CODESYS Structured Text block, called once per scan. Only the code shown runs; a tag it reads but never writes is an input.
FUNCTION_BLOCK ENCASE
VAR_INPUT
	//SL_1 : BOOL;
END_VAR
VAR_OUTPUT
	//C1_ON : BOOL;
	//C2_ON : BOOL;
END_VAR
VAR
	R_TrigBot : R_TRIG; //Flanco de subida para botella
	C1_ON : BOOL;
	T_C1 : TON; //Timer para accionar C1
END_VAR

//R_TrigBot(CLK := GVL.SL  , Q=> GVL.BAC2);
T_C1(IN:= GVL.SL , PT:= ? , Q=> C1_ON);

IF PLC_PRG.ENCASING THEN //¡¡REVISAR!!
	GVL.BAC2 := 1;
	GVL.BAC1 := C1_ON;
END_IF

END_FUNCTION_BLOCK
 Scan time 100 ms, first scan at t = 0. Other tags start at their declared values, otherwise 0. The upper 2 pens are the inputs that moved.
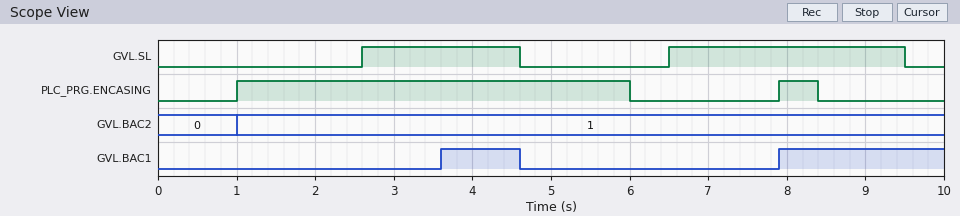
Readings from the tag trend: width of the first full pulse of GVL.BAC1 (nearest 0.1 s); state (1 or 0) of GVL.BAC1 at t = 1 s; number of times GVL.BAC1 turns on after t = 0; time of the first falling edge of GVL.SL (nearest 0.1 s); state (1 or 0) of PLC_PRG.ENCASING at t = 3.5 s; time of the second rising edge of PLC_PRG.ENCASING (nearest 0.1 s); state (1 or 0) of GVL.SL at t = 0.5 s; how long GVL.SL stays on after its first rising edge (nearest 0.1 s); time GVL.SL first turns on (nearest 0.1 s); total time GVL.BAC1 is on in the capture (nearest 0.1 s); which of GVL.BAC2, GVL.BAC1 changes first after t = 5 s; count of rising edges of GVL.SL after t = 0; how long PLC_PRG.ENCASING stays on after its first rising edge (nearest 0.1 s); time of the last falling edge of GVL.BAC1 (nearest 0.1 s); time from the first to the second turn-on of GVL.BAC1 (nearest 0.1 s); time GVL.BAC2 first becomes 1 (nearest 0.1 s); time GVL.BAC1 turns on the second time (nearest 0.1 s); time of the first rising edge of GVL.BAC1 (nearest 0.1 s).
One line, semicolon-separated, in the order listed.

1.0 s; 0; 2; 4.6 s; 1; 7.9 s; 0; 2.0 s; 2.6 s; 3.1 s; GVL.BAC1; 2; 5.0 s; 4.6 s; 4.3 s; 1.0 s; 7.9 s; 3.6 s
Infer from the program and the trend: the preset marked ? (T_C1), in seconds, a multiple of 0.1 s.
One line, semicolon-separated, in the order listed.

1.0 s
